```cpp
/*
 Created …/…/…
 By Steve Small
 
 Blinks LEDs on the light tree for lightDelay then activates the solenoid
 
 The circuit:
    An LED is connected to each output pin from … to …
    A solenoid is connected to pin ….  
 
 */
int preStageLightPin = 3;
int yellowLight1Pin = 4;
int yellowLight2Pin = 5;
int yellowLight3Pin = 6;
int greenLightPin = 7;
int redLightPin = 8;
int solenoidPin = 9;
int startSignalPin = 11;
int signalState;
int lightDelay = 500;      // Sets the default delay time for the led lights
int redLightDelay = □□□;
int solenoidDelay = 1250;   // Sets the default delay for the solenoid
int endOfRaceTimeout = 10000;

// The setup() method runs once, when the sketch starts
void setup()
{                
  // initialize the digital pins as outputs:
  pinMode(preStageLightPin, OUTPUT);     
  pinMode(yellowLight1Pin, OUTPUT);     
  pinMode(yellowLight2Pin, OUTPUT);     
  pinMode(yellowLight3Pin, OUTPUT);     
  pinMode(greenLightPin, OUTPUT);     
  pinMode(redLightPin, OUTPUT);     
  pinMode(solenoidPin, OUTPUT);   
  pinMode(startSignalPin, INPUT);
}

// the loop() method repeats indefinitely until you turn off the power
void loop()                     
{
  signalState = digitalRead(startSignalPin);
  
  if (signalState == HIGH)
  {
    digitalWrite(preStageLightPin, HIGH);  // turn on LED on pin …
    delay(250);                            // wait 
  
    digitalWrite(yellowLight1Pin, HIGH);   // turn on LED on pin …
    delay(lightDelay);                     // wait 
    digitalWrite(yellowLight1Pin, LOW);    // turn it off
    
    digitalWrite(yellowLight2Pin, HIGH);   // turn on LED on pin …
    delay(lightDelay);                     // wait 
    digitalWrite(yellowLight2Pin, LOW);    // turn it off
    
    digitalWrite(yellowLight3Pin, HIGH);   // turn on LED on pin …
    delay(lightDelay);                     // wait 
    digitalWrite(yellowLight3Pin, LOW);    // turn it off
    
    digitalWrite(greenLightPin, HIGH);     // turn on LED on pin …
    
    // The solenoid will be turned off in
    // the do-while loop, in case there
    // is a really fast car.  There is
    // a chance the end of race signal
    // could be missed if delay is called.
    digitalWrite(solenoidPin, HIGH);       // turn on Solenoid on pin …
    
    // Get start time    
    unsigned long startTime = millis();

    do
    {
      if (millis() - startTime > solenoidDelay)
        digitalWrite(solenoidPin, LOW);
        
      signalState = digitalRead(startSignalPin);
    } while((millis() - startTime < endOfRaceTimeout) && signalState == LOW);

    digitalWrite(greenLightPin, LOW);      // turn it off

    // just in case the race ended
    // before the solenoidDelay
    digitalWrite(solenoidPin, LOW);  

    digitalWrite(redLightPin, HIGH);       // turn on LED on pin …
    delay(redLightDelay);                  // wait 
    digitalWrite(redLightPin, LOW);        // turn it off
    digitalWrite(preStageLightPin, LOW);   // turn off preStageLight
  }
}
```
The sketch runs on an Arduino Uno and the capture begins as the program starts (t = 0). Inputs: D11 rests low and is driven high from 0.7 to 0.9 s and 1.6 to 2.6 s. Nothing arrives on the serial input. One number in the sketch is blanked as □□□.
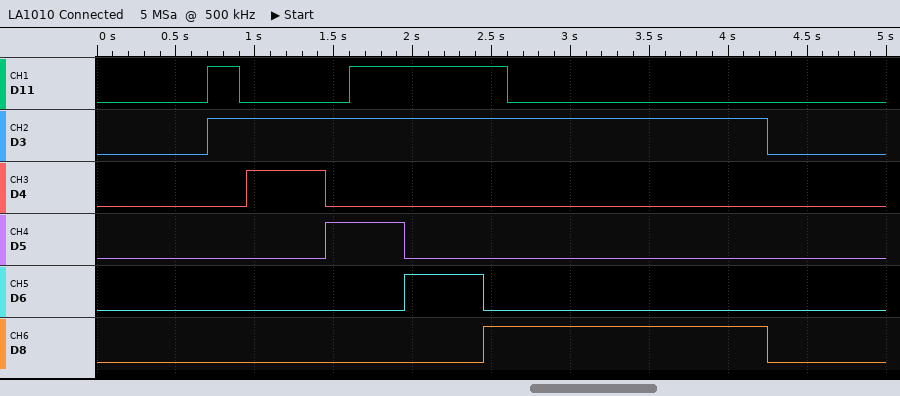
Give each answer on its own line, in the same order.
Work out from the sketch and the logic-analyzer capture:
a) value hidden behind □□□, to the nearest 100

1800
